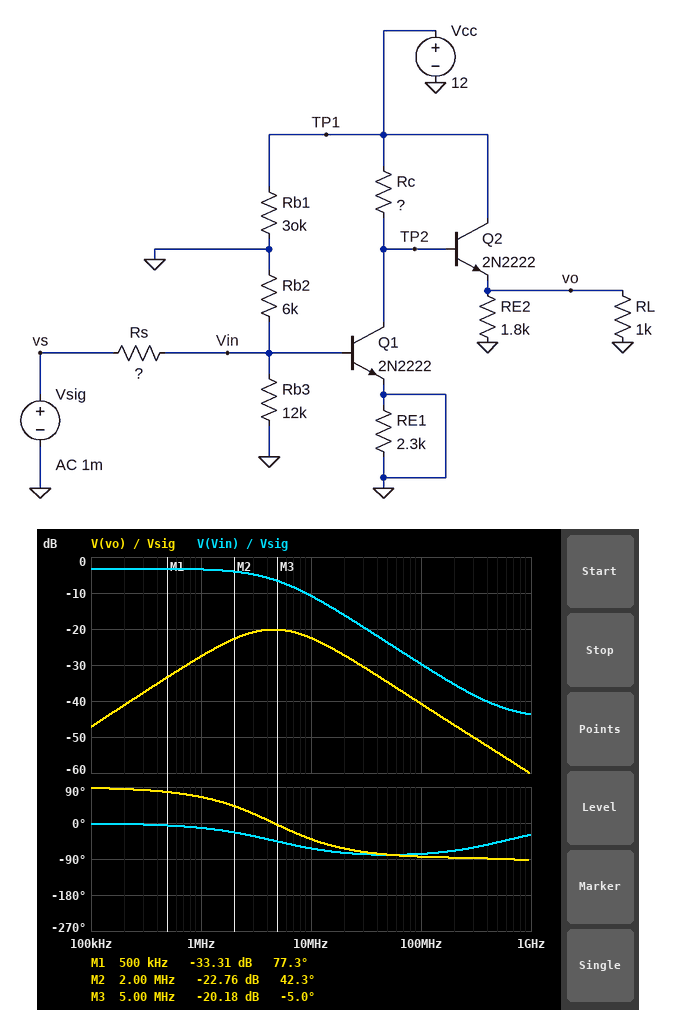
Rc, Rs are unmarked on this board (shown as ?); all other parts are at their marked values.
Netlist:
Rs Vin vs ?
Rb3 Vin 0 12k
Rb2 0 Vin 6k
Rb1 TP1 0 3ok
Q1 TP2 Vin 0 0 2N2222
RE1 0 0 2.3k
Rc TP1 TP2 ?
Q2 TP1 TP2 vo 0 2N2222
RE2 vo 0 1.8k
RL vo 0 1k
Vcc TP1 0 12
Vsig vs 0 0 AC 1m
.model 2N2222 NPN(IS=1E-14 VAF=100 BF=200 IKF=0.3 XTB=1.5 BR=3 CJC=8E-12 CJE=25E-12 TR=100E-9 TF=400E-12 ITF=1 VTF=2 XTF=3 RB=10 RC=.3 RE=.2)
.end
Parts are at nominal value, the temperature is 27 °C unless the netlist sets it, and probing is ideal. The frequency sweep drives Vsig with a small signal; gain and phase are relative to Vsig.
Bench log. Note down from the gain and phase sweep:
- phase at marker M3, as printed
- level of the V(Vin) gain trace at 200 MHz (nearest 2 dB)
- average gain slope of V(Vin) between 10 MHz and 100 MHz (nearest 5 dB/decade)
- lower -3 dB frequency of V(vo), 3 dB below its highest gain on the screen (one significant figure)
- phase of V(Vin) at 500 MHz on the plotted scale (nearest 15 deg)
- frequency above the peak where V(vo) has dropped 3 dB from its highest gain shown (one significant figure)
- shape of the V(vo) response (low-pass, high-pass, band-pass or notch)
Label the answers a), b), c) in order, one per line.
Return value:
a) -5.0 deg
b) -36 dB
c) -20 dB/decade
d) 2 MHz
e) -45 deg
f) 10 MHz
g) band-pass
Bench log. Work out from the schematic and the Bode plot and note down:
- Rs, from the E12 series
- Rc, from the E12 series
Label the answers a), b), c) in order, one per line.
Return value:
a) 1.8 kΩ
b) 3.3 kΩ
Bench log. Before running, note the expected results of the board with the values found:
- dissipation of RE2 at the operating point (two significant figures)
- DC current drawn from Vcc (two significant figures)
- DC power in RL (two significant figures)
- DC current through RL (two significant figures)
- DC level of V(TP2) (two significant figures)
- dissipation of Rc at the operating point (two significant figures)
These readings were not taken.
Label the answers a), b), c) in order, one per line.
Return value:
a) 67 mW
b) 4.0 A
c) 120 mW
d) 11 mA
e) 12 V
f) 26 µW
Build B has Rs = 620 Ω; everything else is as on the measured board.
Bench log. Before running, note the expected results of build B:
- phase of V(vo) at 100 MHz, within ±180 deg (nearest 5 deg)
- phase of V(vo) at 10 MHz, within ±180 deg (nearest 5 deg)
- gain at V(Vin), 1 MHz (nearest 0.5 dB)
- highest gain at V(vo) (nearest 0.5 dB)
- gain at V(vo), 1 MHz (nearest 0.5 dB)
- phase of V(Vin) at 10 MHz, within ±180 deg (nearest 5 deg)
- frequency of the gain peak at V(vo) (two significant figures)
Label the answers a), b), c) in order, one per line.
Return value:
a) -80 deg
b) -20 deg
c) -1.5 dB
d) -15.5 dB
e) -25.5 dB
f) -40 deg
g) 6.9 MHz
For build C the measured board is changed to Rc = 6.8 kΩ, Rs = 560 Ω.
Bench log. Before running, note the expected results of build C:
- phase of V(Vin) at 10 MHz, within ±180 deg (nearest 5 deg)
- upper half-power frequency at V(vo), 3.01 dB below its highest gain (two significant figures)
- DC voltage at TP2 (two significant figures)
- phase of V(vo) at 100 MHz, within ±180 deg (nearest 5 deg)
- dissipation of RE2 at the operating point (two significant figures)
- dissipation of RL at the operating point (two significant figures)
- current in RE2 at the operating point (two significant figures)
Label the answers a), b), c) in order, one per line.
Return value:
a) -40 deg
b) 16 MHz
c) 11 V
d) -80 deg
e) 63 mW
f) 110 mW
g) 5.9 mA
